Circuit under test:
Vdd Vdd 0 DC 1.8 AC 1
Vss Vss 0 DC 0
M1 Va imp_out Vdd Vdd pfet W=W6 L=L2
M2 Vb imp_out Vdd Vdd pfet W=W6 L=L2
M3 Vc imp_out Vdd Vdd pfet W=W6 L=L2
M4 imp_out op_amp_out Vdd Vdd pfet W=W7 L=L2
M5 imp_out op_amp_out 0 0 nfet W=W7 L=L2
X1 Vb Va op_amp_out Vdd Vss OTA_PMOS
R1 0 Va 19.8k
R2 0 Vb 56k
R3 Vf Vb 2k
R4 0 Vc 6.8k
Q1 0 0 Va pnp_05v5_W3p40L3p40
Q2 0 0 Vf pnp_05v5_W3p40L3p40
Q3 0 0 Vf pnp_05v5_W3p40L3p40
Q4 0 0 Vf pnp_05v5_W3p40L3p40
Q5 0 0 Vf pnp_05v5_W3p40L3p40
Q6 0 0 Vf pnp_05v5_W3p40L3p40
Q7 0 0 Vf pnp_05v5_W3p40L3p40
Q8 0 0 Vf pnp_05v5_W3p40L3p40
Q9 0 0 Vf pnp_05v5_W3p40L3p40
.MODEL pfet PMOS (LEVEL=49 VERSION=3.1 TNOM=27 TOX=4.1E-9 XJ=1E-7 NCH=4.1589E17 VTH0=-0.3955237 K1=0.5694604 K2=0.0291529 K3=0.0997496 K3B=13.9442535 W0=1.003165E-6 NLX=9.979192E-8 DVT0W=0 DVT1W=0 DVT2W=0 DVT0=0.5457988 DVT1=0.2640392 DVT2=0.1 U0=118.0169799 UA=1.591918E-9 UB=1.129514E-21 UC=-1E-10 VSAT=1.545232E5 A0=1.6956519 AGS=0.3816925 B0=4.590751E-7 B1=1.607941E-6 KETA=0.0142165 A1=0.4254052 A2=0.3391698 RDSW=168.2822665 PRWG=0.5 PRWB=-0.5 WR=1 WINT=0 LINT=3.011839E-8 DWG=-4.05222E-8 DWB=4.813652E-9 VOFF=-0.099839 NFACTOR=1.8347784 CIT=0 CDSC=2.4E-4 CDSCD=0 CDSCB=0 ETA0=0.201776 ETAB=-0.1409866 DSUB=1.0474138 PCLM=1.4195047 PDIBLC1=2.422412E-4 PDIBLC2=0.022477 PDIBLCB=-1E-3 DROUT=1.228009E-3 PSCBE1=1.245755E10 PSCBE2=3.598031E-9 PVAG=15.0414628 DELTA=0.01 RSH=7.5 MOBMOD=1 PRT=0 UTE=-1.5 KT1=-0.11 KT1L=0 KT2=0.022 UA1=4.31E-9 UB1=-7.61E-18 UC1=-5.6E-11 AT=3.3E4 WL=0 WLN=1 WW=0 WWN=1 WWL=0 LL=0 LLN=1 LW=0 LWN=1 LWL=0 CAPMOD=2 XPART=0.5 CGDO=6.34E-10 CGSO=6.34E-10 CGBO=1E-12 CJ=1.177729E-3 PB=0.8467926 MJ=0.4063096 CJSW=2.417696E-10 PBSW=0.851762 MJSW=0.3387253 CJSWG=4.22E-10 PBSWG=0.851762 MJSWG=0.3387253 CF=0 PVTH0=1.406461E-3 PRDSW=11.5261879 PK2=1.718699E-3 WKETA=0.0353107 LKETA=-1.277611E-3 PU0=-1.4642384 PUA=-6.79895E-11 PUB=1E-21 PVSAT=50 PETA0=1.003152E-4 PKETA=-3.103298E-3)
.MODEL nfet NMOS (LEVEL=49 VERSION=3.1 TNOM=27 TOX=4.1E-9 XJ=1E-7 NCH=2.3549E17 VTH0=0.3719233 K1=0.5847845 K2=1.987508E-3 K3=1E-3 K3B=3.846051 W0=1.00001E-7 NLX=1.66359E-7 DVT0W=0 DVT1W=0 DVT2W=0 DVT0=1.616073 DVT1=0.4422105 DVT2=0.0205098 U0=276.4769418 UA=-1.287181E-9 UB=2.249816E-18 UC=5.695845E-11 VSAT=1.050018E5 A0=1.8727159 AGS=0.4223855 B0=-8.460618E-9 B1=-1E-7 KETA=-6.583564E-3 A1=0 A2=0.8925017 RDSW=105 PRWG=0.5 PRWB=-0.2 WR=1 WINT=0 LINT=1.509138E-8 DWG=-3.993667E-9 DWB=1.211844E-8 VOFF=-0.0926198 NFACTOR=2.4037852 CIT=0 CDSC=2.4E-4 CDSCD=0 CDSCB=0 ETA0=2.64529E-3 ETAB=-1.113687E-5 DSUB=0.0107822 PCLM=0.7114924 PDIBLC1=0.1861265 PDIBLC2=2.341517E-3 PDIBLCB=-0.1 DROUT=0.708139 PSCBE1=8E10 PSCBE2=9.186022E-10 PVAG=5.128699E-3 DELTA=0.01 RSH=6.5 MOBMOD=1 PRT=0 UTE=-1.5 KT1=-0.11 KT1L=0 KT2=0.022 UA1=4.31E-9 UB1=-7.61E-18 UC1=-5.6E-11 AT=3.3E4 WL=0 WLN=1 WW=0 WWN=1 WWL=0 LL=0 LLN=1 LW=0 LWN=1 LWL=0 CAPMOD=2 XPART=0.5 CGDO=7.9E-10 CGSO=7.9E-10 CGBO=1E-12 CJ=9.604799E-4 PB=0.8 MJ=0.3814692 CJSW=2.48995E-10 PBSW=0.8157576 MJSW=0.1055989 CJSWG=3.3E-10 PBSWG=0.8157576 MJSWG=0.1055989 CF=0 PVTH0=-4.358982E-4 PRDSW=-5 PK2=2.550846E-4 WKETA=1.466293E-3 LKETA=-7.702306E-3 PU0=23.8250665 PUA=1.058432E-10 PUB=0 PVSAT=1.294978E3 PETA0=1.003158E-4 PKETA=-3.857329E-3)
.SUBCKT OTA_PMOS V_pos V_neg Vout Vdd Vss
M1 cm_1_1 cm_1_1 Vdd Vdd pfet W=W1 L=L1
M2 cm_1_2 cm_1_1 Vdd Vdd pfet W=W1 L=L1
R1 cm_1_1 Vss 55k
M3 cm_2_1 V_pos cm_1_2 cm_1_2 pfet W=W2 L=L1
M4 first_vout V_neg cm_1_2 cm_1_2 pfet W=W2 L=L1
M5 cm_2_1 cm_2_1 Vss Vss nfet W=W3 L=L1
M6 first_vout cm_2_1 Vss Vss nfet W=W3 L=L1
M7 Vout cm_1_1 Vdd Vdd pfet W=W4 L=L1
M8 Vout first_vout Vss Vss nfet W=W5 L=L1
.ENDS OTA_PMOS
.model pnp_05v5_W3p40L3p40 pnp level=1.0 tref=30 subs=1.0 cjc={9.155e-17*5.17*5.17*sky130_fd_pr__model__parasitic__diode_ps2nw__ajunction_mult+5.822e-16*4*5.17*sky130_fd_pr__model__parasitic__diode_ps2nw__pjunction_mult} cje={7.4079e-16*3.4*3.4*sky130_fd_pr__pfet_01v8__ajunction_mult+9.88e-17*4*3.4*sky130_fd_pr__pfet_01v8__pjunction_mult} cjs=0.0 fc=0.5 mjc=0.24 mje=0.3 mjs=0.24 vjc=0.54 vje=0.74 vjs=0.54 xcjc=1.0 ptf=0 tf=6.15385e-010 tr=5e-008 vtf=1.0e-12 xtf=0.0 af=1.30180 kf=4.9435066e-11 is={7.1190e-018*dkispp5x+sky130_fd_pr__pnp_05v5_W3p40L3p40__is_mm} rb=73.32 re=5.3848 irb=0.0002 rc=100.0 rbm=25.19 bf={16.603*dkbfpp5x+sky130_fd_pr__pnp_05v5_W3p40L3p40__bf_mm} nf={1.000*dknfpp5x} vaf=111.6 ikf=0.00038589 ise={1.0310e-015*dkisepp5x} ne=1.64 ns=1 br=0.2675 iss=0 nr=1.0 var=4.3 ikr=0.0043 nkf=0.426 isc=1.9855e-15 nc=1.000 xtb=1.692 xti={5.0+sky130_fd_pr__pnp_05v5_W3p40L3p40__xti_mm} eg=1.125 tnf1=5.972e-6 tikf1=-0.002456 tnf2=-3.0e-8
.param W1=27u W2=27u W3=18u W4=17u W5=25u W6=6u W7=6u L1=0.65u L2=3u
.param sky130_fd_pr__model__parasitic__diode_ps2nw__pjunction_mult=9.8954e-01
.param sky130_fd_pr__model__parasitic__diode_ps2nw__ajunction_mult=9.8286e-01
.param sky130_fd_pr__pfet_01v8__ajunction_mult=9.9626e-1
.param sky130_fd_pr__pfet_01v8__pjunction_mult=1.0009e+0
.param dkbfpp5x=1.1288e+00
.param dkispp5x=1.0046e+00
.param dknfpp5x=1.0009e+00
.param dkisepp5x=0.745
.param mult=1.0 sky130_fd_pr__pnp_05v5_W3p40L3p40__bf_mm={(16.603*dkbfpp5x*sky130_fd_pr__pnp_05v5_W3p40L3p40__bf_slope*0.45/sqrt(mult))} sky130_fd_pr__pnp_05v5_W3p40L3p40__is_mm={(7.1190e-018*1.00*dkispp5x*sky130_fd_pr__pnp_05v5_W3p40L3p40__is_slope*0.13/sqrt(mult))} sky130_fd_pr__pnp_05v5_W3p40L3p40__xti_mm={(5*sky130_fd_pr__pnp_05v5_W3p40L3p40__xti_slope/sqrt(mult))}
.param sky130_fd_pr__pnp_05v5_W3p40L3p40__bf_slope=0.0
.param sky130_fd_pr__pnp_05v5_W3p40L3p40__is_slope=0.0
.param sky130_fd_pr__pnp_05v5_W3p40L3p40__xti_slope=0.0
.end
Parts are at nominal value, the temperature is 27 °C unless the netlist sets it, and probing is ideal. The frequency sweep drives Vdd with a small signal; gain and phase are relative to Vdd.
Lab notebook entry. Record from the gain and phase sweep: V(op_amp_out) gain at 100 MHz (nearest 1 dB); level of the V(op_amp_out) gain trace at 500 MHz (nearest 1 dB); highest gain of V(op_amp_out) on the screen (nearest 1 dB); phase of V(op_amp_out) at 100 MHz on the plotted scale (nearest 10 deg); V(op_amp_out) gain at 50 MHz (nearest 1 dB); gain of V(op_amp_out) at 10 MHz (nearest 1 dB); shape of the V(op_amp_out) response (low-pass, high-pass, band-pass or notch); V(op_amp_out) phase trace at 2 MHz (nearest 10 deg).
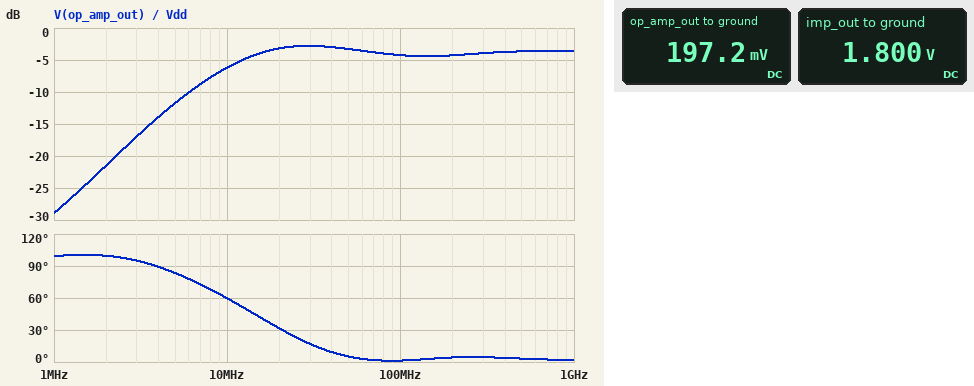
-4 dB
-4 dB
-3 dB
0 deg
-3 dB
-6 dB
high-pass
100 deg
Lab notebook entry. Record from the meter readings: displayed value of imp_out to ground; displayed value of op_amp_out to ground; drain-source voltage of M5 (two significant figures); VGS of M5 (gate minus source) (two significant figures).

1.800 V
197.2 mV
1.8 V
200 mV
